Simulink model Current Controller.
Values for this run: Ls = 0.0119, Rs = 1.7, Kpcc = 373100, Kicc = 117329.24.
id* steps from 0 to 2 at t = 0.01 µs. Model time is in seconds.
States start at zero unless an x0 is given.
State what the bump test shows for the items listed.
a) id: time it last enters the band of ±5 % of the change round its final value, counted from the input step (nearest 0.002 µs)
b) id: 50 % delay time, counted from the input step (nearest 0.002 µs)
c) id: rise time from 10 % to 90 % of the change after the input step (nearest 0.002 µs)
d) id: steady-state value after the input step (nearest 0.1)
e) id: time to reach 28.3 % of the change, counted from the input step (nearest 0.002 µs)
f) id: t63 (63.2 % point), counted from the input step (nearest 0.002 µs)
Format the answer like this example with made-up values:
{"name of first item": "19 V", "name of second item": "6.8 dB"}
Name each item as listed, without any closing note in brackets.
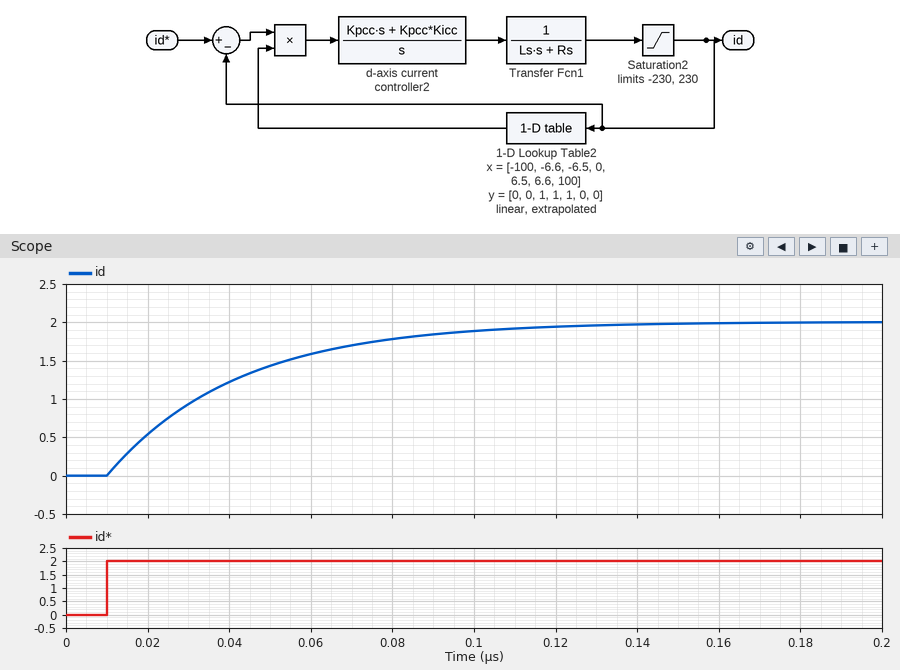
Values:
{"id: time it last enters the band of ±5 % of the change round its final value, counted from the input step": "0.096 µs", "id: 50 % delay time, counted from the input step": "0.022 µs", "id: rise time from 10 % to 90 % of the change after the input step": "0.070 µs", "id: steady-state value after the input step": "2.0", "id: time to reach 28.3 % of the change, counted from the input step": "0.010 µs", "id: t63 (63.2 % point), counted from the input step": "0.032 µs"}
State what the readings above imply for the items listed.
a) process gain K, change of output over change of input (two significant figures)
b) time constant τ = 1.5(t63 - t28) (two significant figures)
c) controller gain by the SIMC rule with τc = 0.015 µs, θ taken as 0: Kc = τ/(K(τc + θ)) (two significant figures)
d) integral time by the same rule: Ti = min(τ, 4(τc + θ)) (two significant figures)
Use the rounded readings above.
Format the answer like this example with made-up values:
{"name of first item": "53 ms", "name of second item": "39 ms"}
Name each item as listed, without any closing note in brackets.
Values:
{"process gain K, change of output over change of input": "1.0", "time constant τ = 1.5(t63 - t28)": "0.033 µs", "controller gain by the SIMC rule with τc = 0.015 µs, θ taken as 0: Kc = τ/(K(τc + θ))": "2.2", "integral time by the same rule: Ti = min(τ, 4(τc + θ))": "0.033 µs"}
